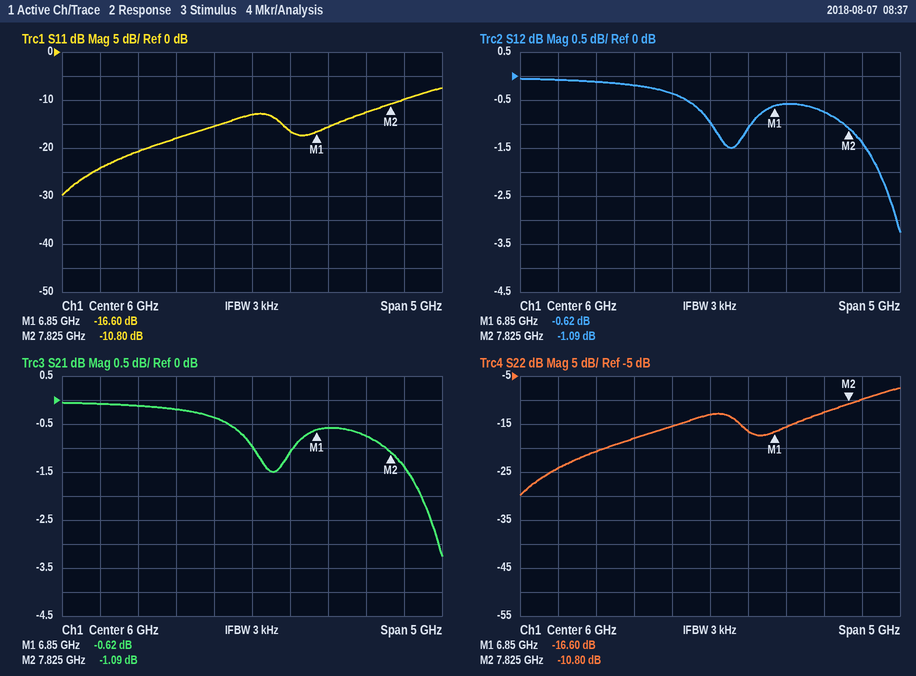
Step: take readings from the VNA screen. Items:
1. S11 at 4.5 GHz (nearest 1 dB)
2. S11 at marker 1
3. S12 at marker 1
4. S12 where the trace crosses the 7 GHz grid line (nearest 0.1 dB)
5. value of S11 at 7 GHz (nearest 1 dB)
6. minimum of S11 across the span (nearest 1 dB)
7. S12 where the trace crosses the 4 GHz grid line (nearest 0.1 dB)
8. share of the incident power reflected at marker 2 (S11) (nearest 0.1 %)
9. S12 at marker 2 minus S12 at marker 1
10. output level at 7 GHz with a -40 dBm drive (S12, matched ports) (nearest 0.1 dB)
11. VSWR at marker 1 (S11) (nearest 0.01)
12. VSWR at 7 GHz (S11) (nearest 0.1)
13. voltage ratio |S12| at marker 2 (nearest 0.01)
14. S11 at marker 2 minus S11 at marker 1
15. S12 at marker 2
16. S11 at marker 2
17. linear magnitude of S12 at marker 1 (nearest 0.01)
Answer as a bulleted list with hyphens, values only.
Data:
- -21 dB
- -16.60 dB
- -0.62 dB
- -0.6 dB
- -16 dB
- -30 dB
- -0.1 dB
- 8.3 %
- -0.47 dB
- -40.6 dBm
- 1.35
- 1.4
- 0.88
- 5.80 dB
- -1.09 dB
- -10.80 dB
- 0.93
